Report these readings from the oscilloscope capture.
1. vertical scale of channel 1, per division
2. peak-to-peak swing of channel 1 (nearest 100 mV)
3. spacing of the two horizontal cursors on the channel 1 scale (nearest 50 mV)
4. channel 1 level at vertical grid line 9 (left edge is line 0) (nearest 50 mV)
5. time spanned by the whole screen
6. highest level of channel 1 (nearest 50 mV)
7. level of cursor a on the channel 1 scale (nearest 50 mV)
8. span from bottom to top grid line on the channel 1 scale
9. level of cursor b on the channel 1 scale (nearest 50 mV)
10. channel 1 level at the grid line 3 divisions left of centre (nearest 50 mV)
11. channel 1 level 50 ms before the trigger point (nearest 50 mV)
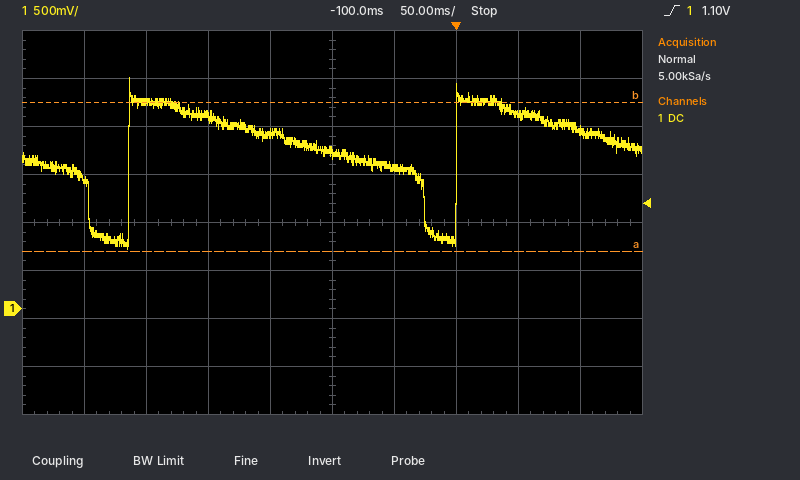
500 mV
1.80 V
1.55 V
1.85 V
500 ms
2.40 V
600 mV
4 V
2.15 V
2.15 V
1.45 V
